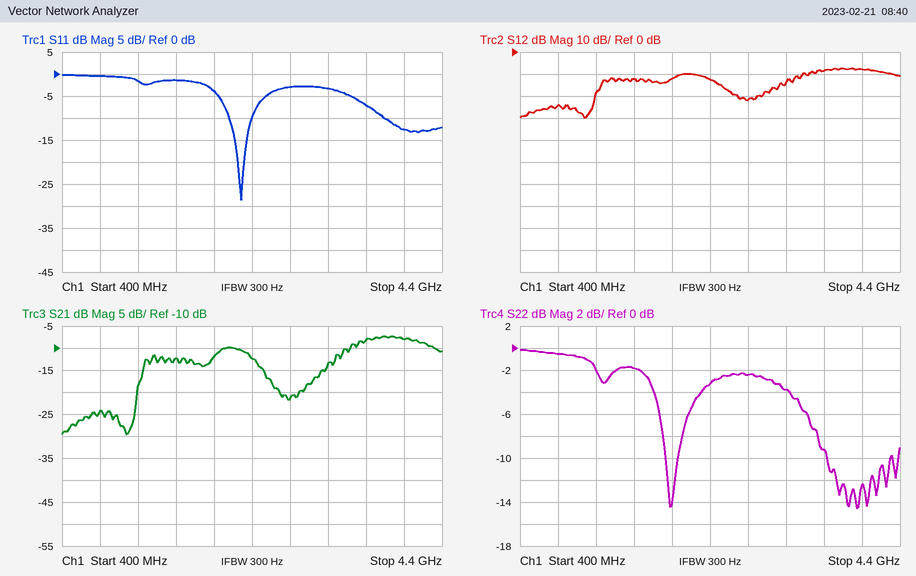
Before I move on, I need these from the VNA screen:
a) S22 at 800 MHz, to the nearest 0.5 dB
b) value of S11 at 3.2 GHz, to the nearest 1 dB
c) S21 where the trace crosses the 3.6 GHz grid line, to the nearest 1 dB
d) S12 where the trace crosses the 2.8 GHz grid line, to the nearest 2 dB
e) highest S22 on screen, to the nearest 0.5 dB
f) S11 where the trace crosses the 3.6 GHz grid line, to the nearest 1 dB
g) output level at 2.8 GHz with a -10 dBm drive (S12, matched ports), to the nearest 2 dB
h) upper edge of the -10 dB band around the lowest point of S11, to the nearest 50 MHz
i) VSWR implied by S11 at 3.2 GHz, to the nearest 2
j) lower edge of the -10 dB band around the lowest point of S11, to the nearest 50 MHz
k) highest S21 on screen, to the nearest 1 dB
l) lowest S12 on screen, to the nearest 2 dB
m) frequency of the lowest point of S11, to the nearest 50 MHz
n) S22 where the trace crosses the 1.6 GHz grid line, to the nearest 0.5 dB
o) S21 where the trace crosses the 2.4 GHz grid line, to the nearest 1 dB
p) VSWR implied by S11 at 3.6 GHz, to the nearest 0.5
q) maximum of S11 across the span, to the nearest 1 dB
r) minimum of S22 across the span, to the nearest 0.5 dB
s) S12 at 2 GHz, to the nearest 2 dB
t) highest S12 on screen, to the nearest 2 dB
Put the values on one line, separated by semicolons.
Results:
-0.5 dB; -3 dB; -8 dB; -22 dB; 0.0 dB; -7 dB; -32 dBm; 2.40 GHz; 6; 2.15 GHz; -7 dB; -30 dB; 2.30 GHz; -2.0 dB; -12 dB; 2.5; 0 dB; -14.5 dB; -12 dB; -8 dB
